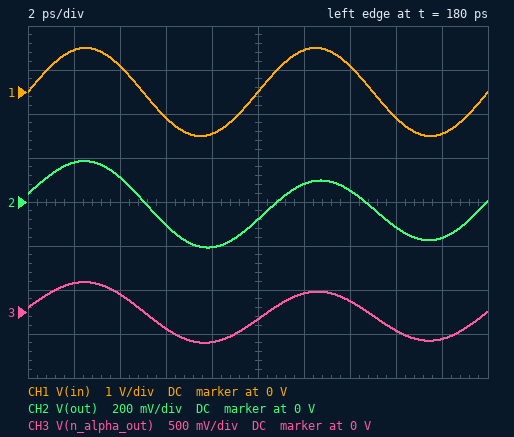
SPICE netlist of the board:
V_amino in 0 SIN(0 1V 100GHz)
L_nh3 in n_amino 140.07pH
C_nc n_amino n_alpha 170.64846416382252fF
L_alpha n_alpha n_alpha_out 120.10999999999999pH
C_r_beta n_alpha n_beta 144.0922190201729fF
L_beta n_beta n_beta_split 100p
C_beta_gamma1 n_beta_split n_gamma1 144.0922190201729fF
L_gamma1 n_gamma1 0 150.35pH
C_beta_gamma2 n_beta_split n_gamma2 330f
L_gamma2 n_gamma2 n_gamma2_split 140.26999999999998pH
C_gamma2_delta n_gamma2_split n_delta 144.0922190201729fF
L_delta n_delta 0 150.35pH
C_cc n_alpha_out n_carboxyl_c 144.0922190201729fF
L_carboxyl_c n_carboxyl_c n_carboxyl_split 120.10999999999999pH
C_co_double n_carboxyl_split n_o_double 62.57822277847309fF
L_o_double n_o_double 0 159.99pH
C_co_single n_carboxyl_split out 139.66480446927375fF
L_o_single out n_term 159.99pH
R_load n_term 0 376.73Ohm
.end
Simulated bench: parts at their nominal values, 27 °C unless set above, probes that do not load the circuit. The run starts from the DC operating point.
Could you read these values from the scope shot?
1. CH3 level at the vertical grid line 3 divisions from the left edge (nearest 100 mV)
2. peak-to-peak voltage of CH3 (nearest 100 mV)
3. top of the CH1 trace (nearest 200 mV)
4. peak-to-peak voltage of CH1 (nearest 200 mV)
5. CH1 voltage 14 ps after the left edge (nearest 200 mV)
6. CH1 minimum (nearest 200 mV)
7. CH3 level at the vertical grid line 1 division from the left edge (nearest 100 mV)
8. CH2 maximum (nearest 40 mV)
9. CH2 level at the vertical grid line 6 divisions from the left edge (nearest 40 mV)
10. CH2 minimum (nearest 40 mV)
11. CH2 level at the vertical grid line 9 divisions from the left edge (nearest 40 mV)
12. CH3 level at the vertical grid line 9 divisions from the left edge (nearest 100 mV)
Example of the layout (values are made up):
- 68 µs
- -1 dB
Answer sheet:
- -200 mV
- 700 mV
- 1.0 V
- 2.0 V
- 600 mV
- -1.0 V
- 300 mV
- 200 mV
- 80 mV
- -200 mV
- -160 mV
- -300 mV
